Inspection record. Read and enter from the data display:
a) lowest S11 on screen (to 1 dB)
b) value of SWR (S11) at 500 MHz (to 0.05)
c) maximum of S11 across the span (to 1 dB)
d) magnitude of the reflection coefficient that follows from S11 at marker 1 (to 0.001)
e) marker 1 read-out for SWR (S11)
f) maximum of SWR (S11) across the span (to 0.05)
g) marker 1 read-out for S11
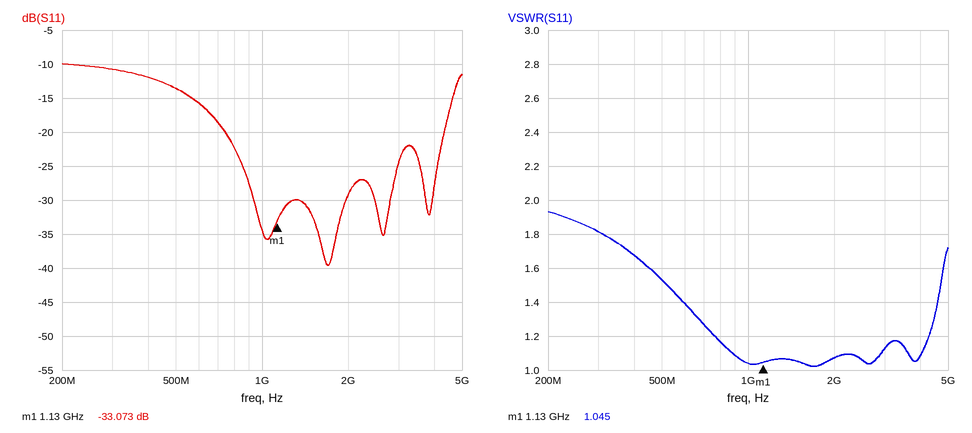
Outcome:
-40 dB
1.55
-10 dB
0.022
1.045
1.95
-33.073 dB
